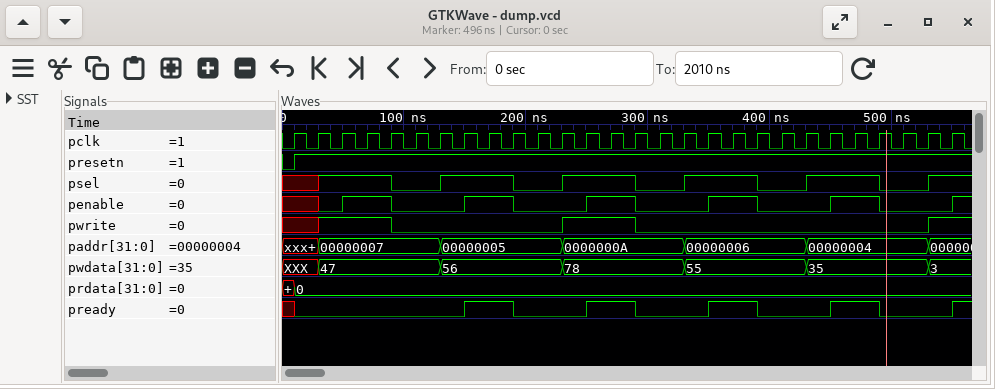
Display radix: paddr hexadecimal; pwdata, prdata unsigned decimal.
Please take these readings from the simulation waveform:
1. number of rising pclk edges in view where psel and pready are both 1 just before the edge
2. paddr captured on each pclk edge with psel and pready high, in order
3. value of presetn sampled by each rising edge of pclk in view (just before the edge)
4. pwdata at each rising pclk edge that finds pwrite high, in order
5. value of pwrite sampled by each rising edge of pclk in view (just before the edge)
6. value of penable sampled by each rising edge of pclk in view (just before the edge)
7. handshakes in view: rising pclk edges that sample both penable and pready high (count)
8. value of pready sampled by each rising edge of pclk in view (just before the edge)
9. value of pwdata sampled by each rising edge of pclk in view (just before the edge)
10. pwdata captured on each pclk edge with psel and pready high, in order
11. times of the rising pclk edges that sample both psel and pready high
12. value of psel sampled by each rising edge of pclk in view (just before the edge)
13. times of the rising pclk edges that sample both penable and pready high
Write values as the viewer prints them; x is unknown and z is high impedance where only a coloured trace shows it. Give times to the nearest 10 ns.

8
00000005, 00000005, 0000000A, 0000000A, 00000006, 00000006, 00000004, 00000004
0 1 1 1 1 1 1 1 1 1 1 1 1 1 1 1 1 1 1 1 1 1 1 1 1 1 1 1
47, 47, 47, 78, 78, 78, 3
x x 1 1 1 0 0 0 0 0 0 0 1 1 1 0 0 0 0 0 0 0 0 0 0 0 0 1
x x 0 1 1 0 0 0 1 1 0 0 0 1 1 0 0 0 1 1 0 0 0 1 1 0 0 0
8
x 0 0 0 0 0 0 0 1 1 0 0 0 1 1 0 0 0 1 1 0 0 0 1 1 0 0 0
XXX, XXX, 47, 47, 47, 47, 47, 56, 56, 56, 56, 56, 78, 78, 78, 78, 78, 55, 55, 55, 55, 55, 35, 35, 35, 35, 35, 3
56, 56, 78, 78, 55, 55, 35, 35
170 ns, 190 ns, 270 ns, 290 ns, 370 ns, 390 ns, 470 ns, 490 ns
x x 1 1 1 0 0 1 1 1 0 0 1 1 1 0 0 1 1 1 0 0 1 1 1 0 0 1
170 ns, 190 ns, 270 ns, 290 ns, 370 ns, 390 ns, 470 ns, 490 ns
